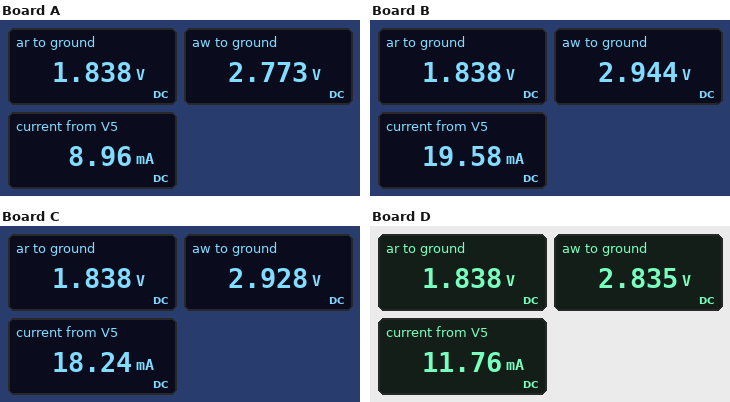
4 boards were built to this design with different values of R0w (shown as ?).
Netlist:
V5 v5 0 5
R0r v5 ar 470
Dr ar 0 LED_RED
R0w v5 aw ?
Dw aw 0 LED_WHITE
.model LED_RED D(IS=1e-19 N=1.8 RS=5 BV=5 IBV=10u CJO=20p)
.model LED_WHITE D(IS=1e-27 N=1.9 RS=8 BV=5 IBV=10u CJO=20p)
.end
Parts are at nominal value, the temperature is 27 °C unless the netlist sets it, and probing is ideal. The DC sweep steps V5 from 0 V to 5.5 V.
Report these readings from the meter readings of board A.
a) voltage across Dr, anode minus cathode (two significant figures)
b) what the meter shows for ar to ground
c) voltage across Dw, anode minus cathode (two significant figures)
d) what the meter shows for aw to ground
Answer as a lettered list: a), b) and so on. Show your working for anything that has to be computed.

a) 1.838 V = 1.8 V
b) 1.838 V
c) 2.773 V = 2.8 V
d) 2.773 V
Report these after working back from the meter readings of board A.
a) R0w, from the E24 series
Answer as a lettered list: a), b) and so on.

a) 1 kΩ
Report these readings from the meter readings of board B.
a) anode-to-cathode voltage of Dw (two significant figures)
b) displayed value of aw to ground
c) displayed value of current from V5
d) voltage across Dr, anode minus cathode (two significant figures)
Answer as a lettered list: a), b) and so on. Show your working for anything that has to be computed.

a) 2.944 V = 2.9 V
b) 2.944 V
c) 19.58 mA
d) 1.838 V = 1.8 V
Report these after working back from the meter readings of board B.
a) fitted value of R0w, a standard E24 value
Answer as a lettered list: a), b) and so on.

a) 160 Ω
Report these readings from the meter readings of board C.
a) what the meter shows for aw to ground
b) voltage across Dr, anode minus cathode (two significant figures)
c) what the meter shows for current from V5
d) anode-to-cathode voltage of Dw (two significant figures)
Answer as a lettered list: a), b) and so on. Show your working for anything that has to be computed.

a) 2.928 V
b) 1.838 V = 1.8 V
c) 18.24 mA
d) 2.928 V = 2.9 V
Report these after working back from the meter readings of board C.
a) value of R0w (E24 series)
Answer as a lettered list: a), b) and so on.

a) 180 Ω
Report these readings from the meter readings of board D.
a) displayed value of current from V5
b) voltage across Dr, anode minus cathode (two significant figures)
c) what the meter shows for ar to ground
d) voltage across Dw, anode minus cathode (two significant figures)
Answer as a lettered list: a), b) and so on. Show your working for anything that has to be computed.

a) 11.76 mA
b) 1.838 V = 1.8 V
c) 1.838 V
d) 2.835 V = 2.8 V
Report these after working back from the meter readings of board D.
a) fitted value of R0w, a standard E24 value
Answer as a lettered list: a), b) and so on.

a) 430 Ω
